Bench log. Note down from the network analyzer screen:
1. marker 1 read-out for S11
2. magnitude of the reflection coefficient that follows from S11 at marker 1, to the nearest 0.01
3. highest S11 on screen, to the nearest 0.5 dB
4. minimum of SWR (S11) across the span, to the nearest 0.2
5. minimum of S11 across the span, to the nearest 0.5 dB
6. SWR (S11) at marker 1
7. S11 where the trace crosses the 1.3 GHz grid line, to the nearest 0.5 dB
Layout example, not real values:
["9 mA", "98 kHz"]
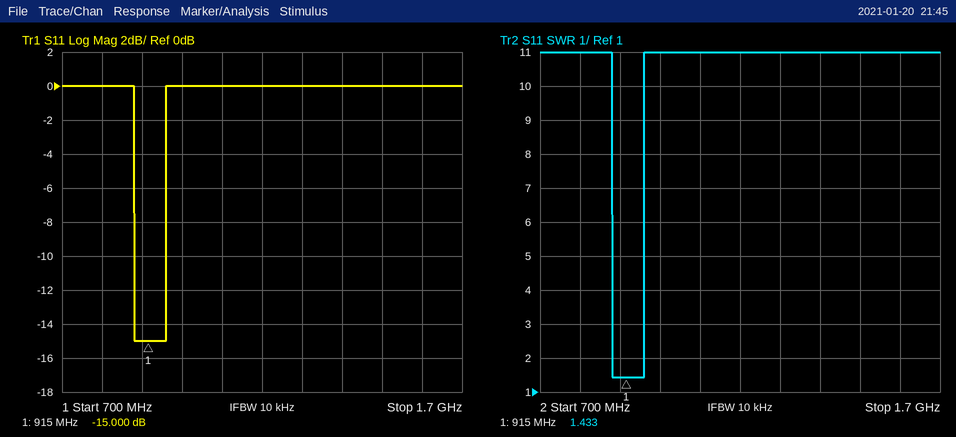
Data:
["-15.000 dB", "0.18", "0.0 dB", "1.4", "-15.0 dB", "1.433", "0.0 dB"]
